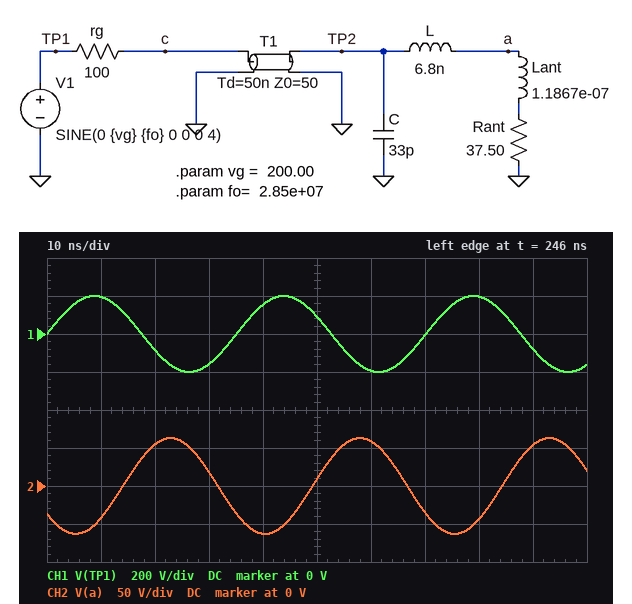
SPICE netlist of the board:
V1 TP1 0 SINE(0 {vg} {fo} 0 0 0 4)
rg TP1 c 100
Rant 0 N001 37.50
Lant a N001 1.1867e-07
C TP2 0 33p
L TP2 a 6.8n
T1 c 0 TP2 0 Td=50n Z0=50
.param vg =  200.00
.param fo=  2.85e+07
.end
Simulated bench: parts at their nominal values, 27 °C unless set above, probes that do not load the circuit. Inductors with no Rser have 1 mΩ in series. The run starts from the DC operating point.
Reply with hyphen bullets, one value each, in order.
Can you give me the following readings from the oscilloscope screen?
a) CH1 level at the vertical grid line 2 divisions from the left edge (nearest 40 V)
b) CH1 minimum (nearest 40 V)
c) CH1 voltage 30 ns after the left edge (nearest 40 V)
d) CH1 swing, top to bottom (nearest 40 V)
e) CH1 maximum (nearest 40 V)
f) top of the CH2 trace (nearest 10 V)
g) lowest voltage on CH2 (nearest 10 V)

- -80 V
- -200 V
- -160 V
- 400 V
- 200 V
- 60 V
- -60 V
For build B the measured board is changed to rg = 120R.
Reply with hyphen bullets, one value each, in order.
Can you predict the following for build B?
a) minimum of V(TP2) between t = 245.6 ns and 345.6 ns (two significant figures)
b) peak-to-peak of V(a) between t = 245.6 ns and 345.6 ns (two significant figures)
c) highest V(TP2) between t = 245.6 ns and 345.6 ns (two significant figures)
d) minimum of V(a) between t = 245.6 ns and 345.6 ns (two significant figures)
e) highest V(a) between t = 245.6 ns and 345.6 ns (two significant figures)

- -56 V
- 110 V
- 56 V
- -55 V
- 55 V
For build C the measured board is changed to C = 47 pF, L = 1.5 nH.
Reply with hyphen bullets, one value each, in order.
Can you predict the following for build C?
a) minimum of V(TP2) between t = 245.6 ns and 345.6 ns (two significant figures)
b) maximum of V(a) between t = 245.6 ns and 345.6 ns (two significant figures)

- -65 V
- 65 V
